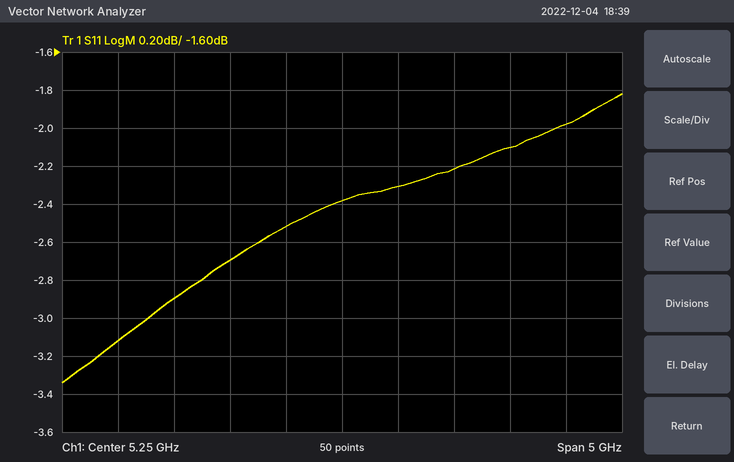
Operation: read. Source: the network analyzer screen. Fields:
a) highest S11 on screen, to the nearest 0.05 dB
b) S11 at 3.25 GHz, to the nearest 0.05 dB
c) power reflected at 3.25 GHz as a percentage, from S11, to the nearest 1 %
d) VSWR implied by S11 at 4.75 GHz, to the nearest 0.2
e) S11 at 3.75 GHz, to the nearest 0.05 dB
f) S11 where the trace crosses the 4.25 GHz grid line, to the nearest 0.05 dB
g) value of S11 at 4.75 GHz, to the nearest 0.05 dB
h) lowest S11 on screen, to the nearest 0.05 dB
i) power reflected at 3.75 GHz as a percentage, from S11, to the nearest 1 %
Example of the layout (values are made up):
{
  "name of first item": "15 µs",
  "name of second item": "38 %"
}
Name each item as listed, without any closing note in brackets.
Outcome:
{
  "highest S11 on screen, to the nearest 0.05 dB": "-1.80 dB",
  "S11 at 3.25 GHz, to the nearest 0.05 dB": "-3.10 dB",
  "power reflected at 3.25 GHz as a percentage, from S11, to the nearest 1 %": "49 %",
  "VSWR implied by S11 at 4.75 GHz, to the nearest 0.2": "7.0",
  "S11 at 3.75 GHz, to the nearest 0.05 dB": "-2.90 dB",
  "S11 where the trace crosses the 4.25 GHz grid line, to the nearest 0.05 dB": "-2.70 dB",
  "value of S11 at 4.75 GHz, to the nearest 0.05 dB": "-2.50 dB",
  "lowest S11 on screen, to the nearest 0.05 dB": "-3.35 dB",
  "power reflected at 3.75 GHz as a percentage, from S11, to the nearest 1 %": "51 %"
}
